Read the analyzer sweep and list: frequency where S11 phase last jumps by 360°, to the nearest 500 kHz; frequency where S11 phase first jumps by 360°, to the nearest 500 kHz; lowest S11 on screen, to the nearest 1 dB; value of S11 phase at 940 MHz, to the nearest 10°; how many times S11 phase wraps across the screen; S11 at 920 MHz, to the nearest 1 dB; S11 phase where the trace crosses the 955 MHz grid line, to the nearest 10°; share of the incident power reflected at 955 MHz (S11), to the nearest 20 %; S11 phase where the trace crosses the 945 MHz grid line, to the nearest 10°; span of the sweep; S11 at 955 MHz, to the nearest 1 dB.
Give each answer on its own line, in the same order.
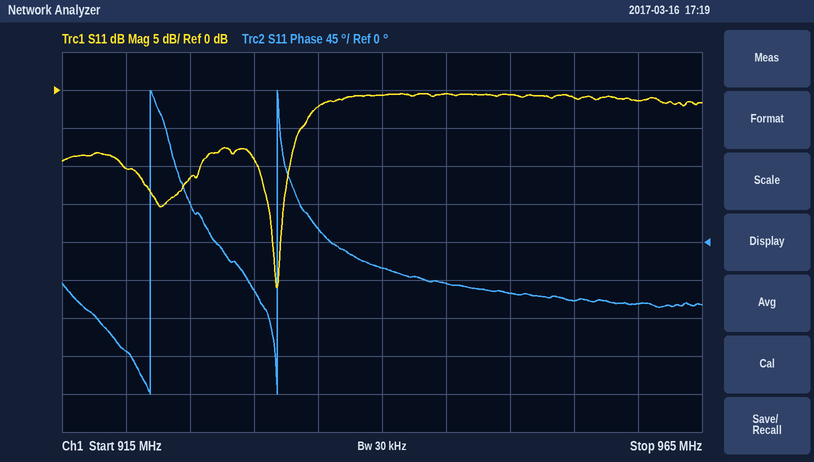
932.0 MHz
922.0 MHz
-26 dB
-30°
2
-10 dB
-70°
80 %
-50°
50 MHz
-1 dB
